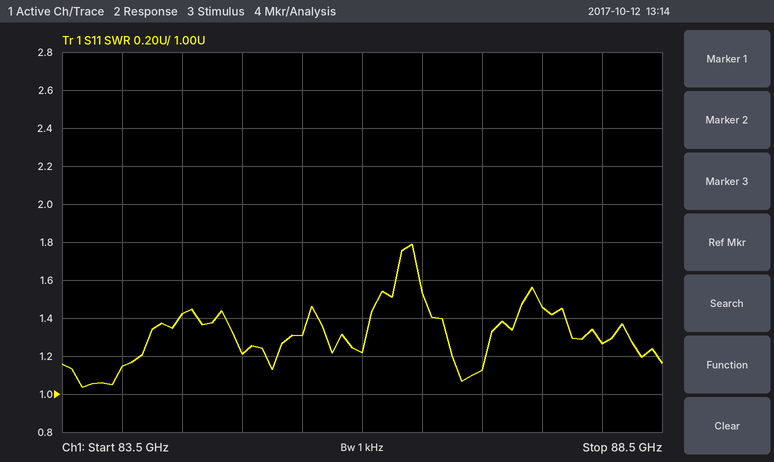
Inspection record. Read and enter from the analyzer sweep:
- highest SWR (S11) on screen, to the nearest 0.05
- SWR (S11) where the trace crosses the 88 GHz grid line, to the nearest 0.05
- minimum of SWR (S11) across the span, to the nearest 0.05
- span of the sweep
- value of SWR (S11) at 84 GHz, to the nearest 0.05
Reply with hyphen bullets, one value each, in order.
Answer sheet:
- 1.80
- 1.25
- 1.05
- 5 GHz
- 1.15
